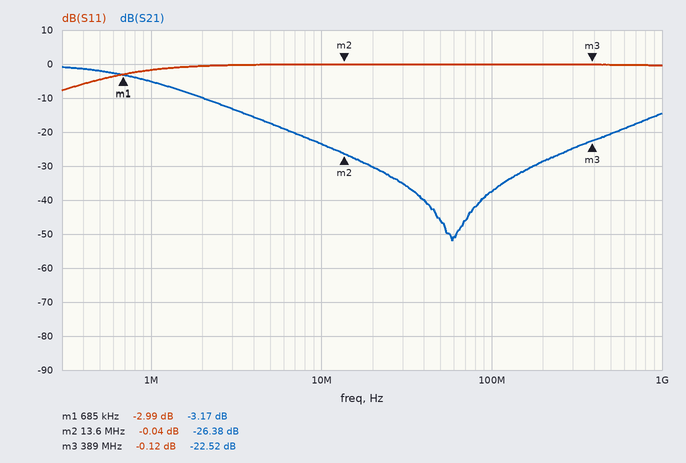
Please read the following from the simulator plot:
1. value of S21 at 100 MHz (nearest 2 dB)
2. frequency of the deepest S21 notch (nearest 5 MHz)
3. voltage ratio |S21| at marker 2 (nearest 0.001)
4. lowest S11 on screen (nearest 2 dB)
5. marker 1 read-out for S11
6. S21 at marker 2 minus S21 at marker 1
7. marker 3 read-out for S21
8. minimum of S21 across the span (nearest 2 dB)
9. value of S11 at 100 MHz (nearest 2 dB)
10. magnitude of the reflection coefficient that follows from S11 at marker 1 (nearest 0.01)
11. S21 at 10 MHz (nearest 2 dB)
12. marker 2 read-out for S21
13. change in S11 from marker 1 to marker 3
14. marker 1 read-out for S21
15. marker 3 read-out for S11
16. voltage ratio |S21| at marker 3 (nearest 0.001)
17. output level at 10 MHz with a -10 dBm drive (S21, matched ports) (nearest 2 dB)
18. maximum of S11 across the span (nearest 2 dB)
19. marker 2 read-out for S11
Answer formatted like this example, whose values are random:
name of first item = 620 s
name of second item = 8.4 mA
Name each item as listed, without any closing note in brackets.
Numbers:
value of S21 at 100 MHz = -38 dB
frequency of the deepest S21 notch = 60 MHz
voltage ratio |S21| at marker 2 = 0.048
lowest S11 on screen = -8 dB
marker 1 read-out for S11 = -2.99 dB
S21 at marker 2 minus S21 at marker 1 = -23.21 dB
marker 3 read-out for S21 = -22.52 dB
minimum of S21 across the span = -52 dB
value of S11 at 100 MHz = 0 dB
magnitude of the reflection coefficient that follows from S11 at marker 1 = 0.71
S21 at 10 MHz = -24 dB
marker 2 read-out for S21 = -26.38 dB
change in S11 from marker 1 to marker 3 = 2.87 dB
marker 1 read-out for S21 = -3.17 dB
marker 3 read-out for S11 = -0.12 dB
voltage ratio |S21| at marker 3 = 0.075
output level at 10 MHz with a -10 dBm drive (S21, matched ports) = -34 dBm
maximum of S11 across the span = 0 dB
marker 2 read-out for S11 = -0.04 dB
